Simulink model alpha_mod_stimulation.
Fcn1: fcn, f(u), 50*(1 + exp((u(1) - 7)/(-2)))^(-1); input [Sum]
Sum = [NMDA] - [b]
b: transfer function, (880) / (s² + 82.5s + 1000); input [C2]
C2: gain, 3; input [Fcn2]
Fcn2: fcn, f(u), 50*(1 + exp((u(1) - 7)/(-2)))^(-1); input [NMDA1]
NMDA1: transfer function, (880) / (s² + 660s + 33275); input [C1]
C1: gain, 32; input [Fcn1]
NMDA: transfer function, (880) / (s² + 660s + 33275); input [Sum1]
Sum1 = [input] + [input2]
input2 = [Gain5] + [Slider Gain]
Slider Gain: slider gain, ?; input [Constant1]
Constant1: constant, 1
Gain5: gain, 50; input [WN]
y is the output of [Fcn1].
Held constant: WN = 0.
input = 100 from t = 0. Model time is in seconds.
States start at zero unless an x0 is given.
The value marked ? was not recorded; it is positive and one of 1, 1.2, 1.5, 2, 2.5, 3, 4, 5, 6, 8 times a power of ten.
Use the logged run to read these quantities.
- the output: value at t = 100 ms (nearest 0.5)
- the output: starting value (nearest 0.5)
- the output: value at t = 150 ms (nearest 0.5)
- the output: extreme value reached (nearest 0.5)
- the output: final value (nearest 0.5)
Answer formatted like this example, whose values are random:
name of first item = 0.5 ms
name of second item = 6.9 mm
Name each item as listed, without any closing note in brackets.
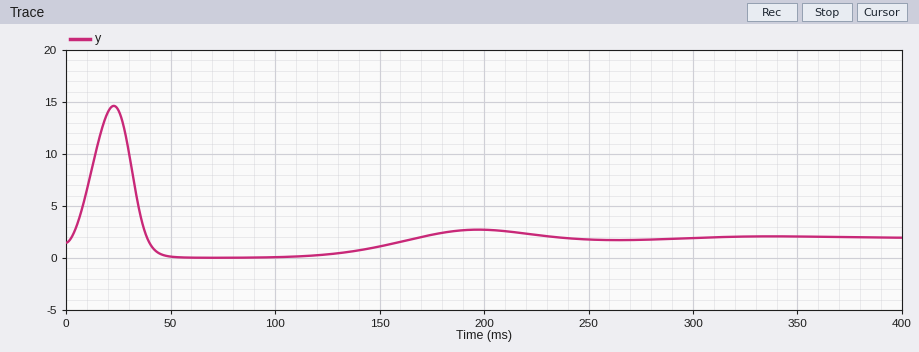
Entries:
the output: value at t = 100 ms = 0.0
the output: starting value = 1.5
the output: value at t = 150 ms = 1.0
the output: extreme value reached = 14.5
the output: final value = 2.0
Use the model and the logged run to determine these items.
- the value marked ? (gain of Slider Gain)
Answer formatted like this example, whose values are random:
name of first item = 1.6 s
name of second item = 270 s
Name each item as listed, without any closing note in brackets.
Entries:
the value marked ? = 250
